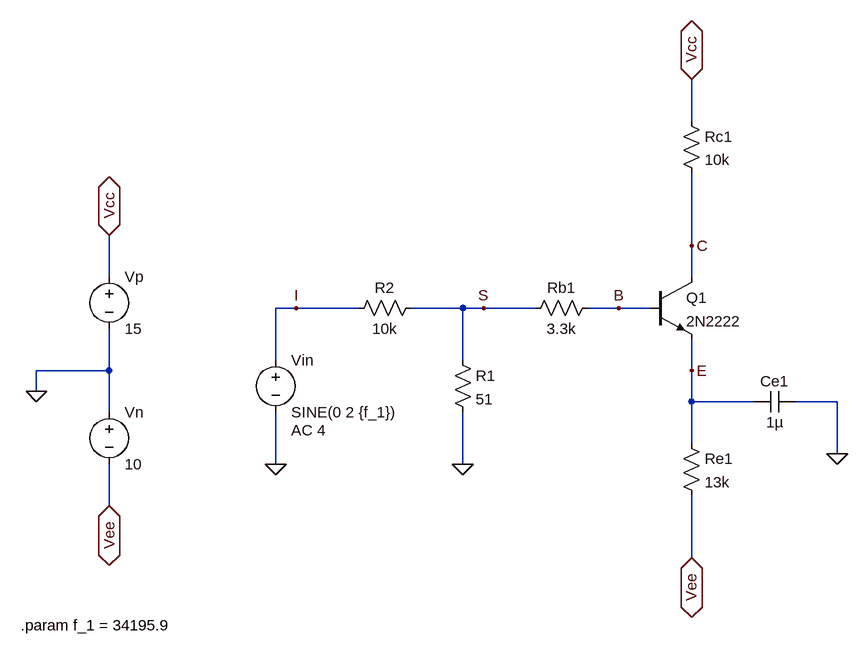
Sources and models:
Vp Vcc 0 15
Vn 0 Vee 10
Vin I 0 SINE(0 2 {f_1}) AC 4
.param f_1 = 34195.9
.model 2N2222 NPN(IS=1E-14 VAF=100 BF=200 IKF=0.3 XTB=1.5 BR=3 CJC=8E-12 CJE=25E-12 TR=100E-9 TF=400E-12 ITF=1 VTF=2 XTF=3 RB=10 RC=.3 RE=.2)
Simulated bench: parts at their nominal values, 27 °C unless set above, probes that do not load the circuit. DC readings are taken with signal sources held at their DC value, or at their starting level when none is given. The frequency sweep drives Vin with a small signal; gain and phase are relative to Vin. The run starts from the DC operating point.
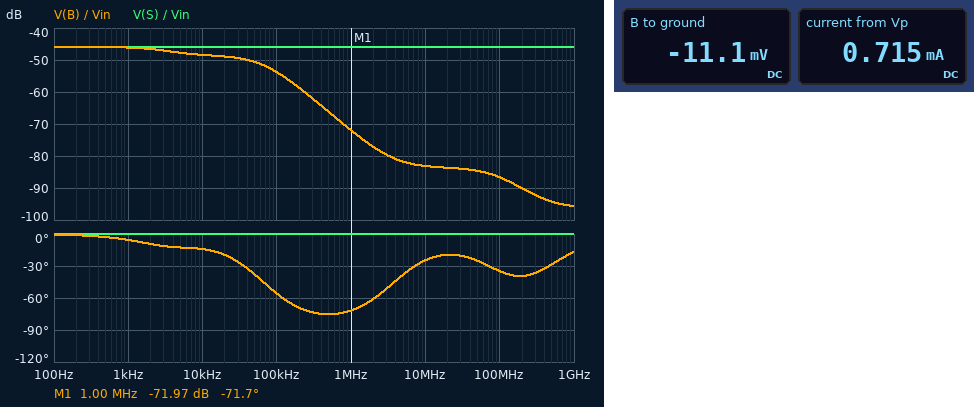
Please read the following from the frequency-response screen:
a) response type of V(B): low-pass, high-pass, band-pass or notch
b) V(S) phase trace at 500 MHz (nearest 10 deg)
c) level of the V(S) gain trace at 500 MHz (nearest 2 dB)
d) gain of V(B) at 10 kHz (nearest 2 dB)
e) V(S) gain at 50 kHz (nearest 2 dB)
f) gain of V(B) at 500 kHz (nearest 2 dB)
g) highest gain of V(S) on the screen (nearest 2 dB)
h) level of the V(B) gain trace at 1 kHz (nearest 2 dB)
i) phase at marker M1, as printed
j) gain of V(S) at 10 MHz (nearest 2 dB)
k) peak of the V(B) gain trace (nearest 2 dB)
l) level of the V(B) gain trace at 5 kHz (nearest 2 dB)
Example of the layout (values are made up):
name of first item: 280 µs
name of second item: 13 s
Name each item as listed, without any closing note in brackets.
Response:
response type of V(B): low-pass, high-pass, band-pass or notch: low-pass
V(S) phase trace at 500 MHz: 0 deg
level of the V(S) gain trace at 500 MHz: -46 dB
gain of V(B) at 10 kHz: -48 dB
V(S) gain at 50 kHz: -46 dB
gain of V(B) at 500 kHz: -66 dB
highest gain of V(S) on the screen: -46 dB
level of the V(B) gain trace at 1 kHz: -46 dB
phase at marker M1, as printed: -71.7 deg
gain of V(S) at 10 MHz: -46 dB
peak of the V(B) gain trace: -46 dB
level of the V(B) gain trace at 5 kHz: -48 dB
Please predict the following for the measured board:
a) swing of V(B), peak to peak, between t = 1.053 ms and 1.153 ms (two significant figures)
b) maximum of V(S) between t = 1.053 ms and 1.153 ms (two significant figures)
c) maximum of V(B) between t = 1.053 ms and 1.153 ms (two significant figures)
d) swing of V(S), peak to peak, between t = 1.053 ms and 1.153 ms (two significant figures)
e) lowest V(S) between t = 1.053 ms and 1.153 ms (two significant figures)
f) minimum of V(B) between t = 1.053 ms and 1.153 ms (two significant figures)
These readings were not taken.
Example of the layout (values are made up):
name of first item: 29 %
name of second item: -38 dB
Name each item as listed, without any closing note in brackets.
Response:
swing of V(B), peak to peak, between t = 1.053 ms and 1.153 ms: 13 mV
maximum of V(S) between t = 1.053 ms and 1.153 ms: 9.9 mV
maximum of V(B) between t = 1.053 ms and 1.153 ms: -4.8 mV
swing of V(S), peak to peak, between t = 1.053 ms and 1.153 ms: 20 mV
lowest V(S) between t = 1.053 ms and 1.153 ms: -10 mV
minimum of V(B) between t = 1.053 ms and 1.153 ms: -18 mV
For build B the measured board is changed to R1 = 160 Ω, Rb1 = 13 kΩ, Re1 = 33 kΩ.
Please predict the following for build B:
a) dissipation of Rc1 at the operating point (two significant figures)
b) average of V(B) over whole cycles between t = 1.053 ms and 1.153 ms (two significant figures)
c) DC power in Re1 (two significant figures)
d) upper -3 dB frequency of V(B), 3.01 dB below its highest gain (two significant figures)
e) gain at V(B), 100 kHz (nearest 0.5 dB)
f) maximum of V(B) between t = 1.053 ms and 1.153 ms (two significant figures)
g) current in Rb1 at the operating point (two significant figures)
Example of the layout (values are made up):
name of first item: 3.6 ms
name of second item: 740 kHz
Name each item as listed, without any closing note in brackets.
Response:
dissipation of Rc1 at the operating point: 800 µW
average of V(B) over whole cycles between t = 1.053 ms and 1.153 ms: -17 mV
DC power in Re1: 2.7 mW
upper -3 dB frequency of V(B), 3.01 dB below its highest gain: 2.2 kHz
gain at V(B), 100 kHz: -47.0 dB
maximum of V(B) between t = 1.053 ms and 1.153 ms: -1.3 mV
current in Rb1 at the operating point: 1.3 µA
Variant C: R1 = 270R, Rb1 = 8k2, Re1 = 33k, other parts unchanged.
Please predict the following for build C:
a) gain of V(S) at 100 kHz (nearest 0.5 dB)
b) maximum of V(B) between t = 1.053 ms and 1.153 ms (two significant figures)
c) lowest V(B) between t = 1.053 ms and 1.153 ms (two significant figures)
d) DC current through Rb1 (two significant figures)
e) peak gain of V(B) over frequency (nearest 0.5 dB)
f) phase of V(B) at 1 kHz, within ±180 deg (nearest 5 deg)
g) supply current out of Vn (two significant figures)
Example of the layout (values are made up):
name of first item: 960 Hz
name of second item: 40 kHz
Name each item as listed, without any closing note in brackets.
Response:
gain of V(S) at 100 kHz: -32.0 dB
maximum of V(B) between t = 1.053 ms and 1.153 ms: 21 mV
lowest V(B) between t = 1.053 ms and 1.153 ms: -53 mV
DC current through Rb1: 1.3 µA
peak gain of V(B) over frequency: -31.5 dB
phase of V(B) at 1 kHz, within ±180 deg: -10 deg
supply current out of Vn: 280 µA
